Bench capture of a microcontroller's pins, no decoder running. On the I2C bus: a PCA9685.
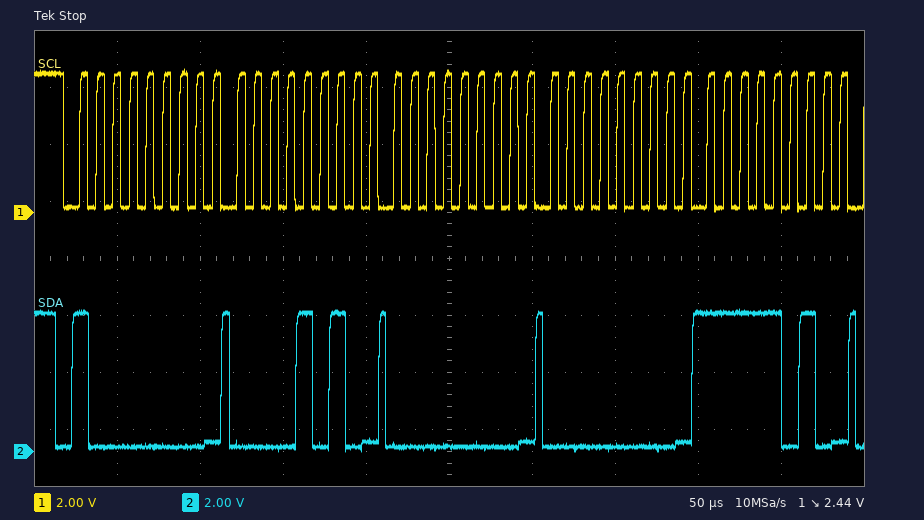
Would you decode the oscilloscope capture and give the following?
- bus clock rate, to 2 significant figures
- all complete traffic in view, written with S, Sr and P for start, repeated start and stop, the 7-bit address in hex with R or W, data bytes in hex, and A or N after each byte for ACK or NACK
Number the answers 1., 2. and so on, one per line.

1. 100 kHz
2. S 40W A 0A A 00 A 00 A FA A
